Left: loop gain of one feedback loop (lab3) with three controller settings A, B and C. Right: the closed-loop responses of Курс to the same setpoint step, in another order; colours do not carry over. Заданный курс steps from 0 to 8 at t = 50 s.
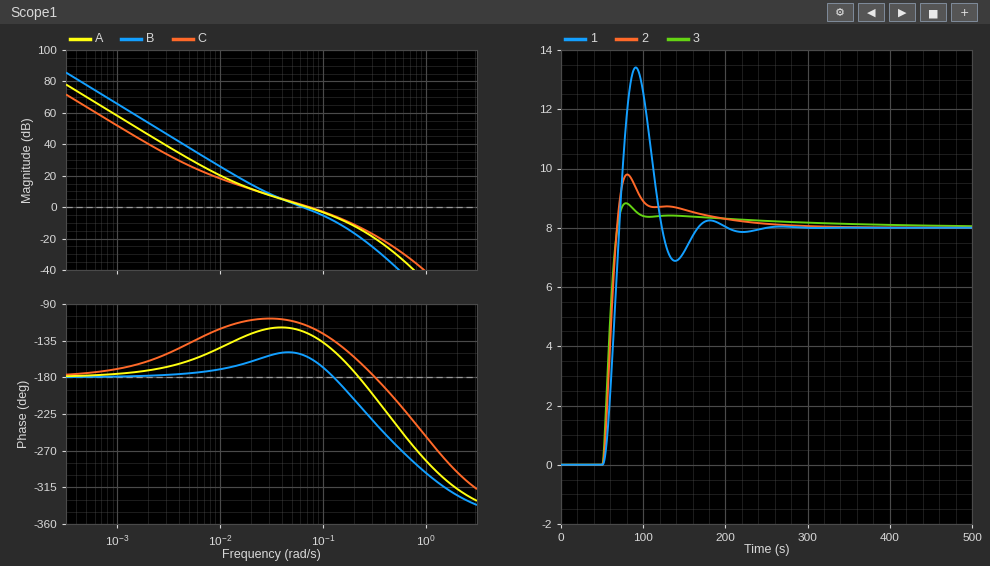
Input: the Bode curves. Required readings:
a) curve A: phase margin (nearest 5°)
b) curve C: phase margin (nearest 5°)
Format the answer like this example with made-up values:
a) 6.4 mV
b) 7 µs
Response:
a) 55°
b) 60°
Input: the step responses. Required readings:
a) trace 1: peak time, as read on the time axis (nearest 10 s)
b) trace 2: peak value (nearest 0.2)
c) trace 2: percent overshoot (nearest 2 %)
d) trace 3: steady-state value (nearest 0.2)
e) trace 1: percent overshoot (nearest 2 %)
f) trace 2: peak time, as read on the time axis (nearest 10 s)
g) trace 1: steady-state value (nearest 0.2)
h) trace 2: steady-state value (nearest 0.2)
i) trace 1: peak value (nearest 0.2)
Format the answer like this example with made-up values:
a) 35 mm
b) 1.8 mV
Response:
a) 90 s
b) 9.8
c) 22 %
d) 8.0
e) 68 %
f) 80 s
g) 8.0
h) 8.0
i) 13.4
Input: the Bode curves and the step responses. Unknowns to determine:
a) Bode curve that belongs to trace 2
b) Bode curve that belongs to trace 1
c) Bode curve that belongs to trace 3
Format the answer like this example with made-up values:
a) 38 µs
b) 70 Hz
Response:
a) A
b) B
c) C
